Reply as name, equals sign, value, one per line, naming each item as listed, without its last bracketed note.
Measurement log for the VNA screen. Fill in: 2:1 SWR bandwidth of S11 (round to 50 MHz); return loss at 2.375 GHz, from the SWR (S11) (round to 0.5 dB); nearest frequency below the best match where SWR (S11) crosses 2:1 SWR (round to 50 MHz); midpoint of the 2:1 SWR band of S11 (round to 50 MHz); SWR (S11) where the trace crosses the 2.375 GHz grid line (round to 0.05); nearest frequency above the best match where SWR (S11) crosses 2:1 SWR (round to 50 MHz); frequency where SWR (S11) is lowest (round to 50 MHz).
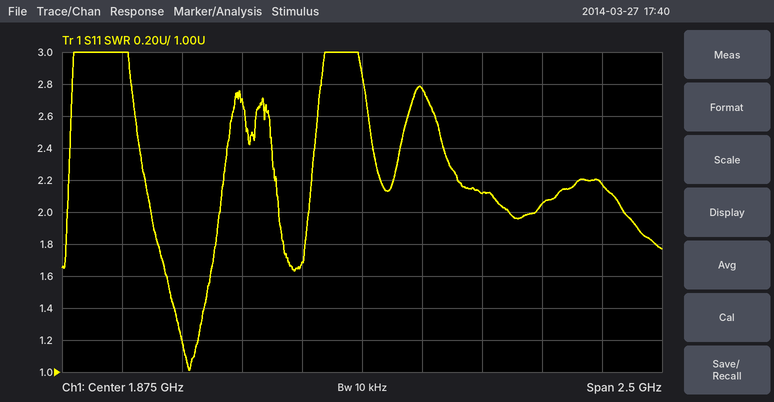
2:1 SWR bandwidth of S11 = 300 MHz
return loss at 2.375 GHz, from the SWR (S11) = 9.0 dB
nearest frequency below the best match where SWR (S11) crosses 2:1 SWR = 1.00 GHz
midpoint of the 2:1 SWR band of S11 = 1.15 GHz
SWR (S11) where the trace crosses the 2.375 GHz grid line = 2.10
nearest frequency above the best match where SWR (S11) crosses 2:1 SWR = 1.30 GHz
frequency where SWR (S11) is lowest = 1.15 GHz
